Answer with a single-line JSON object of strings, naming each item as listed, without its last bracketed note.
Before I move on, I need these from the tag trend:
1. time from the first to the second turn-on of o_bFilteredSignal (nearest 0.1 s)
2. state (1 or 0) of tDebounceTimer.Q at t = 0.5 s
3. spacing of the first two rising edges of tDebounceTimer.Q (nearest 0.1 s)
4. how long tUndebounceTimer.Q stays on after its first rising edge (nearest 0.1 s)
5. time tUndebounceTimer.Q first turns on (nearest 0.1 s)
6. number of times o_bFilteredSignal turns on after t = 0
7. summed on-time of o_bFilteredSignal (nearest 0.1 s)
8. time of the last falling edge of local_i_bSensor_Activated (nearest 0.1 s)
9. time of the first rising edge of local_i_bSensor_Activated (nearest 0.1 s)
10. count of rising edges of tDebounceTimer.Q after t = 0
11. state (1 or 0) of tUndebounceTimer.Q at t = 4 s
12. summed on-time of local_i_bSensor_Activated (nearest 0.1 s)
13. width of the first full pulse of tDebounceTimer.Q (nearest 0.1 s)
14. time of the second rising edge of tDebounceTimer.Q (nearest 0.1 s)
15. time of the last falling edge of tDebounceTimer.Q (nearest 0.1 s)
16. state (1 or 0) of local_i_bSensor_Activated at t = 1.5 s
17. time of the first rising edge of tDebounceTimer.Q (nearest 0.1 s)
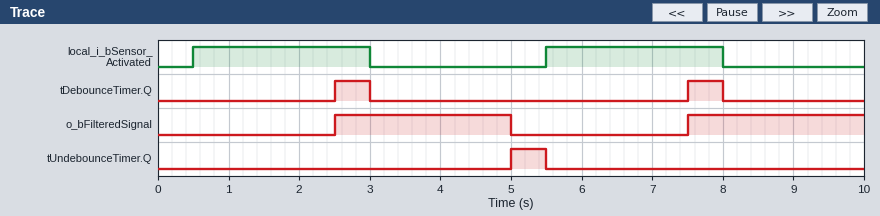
{"time from the first to the second turn-on of o_bFilteredSignal": "5.0 s", "state (1 or 0) of tDebounceTimer.Q at t = 0.5 s": "0", "spacing of the first two rising edges of tDebounceTimer.Q": "5.0 s", "how long tUndebounceTimer.Q stays on after its first rising edge": "0.5 s", "time tUndebounceTimer.Q first turns on": "5.0 s", "number of times o_bFilteredSignal turns on after t = 0": "2", "summed on-time of o_bFilteredSignal": "5.0 s", "time of the last falling edge of local_i_bSensor_Activated": "8.0 s", "time of the first rising edge of local_i_bSensor_Activated": "0.5 s", "count of rising edges of tDebounceTimer.Q after t = 0": "2", "state (1 or 0) of tUndebounceTimer.Q at t = 4 s": "0", "summed on-time of local_i_bSensor_Activated": "5.0 s", "width of the first full pulse of tDebounceTimer.Q": "0.5 s", "time of the second rising edge of tDebounceTimer.Q": "7.5 s", "time of the last falling edge of tDebounceTimer.Q": "8.0 s", "state (1 or 0) of local_i_bSensor_Activated at t = 1.5 s": "1", "time of the first rising edge of tDebounceTimer.Q": "2.5 s"}
